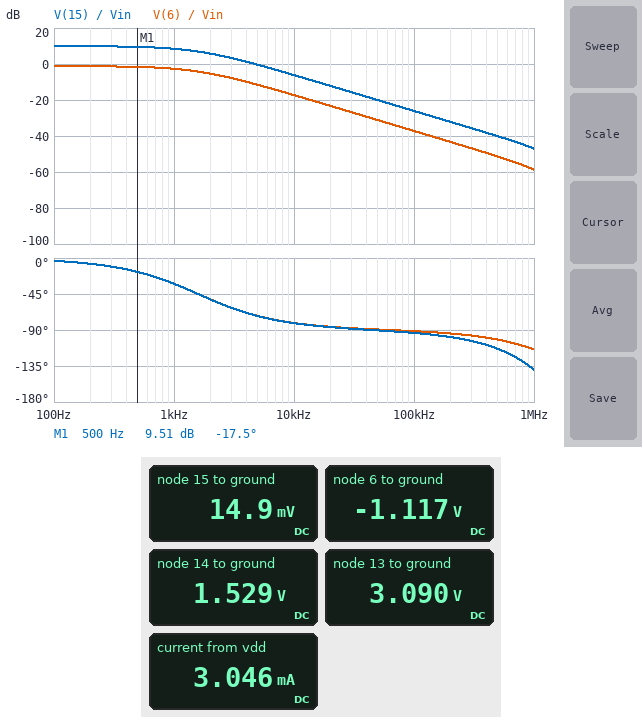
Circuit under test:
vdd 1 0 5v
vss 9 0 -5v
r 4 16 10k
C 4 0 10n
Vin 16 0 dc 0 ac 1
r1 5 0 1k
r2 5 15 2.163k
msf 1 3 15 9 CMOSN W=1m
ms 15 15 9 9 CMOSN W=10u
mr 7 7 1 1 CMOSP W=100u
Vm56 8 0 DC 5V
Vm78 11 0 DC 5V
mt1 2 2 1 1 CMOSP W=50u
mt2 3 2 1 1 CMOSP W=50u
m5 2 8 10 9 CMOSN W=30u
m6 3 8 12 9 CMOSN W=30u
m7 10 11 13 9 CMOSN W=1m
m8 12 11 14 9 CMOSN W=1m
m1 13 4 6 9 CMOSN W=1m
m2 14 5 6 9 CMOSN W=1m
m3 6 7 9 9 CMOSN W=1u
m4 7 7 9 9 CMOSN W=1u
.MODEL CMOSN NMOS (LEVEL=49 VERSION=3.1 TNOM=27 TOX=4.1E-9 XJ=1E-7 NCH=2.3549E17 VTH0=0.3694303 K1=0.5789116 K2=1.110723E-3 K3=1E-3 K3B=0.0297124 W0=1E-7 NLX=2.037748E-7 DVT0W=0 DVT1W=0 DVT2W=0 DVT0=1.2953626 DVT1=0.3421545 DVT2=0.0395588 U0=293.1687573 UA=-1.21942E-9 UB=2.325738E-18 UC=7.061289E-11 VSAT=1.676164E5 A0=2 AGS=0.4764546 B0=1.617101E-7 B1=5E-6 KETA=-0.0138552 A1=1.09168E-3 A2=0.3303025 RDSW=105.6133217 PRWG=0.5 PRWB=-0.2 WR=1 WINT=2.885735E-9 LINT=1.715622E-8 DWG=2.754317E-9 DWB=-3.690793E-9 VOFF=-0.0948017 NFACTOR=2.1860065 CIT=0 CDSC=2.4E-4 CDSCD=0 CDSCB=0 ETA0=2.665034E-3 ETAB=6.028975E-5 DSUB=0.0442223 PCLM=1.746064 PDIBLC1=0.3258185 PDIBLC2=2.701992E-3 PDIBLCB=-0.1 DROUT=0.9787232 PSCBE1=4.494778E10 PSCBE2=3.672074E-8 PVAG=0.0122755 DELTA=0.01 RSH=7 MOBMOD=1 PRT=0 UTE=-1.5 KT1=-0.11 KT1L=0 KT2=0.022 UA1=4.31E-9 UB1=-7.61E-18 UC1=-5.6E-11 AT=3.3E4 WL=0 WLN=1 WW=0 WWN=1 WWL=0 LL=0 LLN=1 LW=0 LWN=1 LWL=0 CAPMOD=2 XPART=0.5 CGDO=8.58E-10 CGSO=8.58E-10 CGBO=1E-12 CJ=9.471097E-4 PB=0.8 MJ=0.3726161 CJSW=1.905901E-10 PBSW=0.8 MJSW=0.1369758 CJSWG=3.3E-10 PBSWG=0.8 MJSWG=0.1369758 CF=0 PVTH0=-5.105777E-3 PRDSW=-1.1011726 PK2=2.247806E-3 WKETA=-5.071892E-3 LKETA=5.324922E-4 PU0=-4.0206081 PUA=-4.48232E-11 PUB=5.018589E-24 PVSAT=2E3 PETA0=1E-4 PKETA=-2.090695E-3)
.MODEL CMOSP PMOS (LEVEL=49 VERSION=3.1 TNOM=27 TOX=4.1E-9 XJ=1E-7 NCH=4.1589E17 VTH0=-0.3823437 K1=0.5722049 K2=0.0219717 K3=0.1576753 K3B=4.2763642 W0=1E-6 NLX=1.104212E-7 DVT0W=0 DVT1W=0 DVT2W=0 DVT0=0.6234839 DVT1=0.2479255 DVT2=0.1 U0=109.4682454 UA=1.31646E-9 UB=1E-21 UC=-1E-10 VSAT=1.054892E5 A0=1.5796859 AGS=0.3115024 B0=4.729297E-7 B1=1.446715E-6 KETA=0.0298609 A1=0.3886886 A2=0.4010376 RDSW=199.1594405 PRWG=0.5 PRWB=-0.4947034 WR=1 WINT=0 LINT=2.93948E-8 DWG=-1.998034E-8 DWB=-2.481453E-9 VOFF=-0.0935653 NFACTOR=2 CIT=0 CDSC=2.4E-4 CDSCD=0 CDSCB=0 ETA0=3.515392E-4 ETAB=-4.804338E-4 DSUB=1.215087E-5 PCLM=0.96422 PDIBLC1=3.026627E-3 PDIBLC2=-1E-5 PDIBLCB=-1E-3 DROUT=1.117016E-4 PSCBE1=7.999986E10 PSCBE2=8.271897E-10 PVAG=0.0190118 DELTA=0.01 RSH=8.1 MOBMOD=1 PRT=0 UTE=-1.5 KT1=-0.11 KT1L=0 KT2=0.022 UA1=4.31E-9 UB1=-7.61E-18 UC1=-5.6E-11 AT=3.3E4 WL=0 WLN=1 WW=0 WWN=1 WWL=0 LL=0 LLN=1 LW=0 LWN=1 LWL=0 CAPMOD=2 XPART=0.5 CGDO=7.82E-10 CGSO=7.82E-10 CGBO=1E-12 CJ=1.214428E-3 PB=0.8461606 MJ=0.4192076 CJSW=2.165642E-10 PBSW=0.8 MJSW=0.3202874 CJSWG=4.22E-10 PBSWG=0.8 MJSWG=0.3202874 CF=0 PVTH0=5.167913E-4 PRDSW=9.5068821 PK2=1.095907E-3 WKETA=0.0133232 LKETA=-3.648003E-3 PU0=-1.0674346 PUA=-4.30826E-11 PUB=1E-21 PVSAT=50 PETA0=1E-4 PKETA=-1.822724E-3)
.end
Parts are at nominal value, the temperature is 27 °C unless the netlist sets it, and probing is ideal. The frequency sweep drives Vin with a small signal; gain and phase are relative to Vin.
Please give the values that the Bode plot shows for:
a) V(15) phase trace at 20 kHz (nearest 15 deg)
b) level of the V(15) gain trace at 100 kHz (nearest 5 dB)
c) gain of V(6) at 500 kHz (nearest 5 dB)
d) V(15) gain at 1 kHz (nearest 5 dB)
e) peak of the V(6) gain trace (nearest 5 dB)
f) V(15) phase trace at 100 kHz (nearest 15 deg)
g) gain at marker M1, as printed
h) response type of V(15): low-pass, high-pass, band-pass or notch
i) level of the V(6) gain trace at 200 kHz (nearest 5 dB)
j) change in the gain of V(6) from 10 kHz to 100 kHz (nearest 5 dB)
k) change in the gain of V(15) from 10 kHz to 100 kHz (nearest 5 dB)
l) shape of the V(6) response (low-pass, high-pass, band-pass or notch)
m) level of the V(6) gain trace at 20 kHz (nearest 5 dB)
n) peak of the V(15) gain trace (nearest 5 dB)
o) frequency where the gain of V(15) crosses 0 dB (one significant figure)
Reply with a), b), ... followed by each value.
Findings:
a) -90 deg
b) -25 dB
c) -50 dB
d) 10 dB
e) 0 dB
f) -90 deg
g) 9.51 dB
h) low-pass
i) -45 dB
j) -20 dB
k) -20 dB
l) low-pass
m) -25 dB
n) 10 dB
o) 5 kHz
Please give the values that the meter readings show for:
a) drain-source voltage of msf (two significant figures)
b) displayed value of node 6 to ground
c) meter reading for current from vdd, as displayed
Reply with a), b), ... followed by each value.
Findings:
a) 5.0 V
b) -1.117 V
c) 3.046 mA
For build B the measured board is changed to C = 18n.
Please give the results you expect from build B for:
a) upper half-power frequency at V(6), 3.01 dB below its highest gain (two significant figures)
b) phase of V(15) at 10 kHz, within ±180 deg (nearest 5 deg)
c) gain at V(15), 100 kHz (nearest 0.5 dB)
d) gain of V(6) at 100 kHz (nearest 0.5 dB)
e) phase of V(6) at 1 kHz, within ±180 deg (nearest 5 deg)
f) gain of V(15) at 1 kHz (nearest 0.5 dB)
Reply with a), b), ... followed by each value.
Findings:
a) 880 Hz
b) -85 deg
c) -31.0 dB
d) -42.5 dB
e) -50 deg
f) 6.5 dB
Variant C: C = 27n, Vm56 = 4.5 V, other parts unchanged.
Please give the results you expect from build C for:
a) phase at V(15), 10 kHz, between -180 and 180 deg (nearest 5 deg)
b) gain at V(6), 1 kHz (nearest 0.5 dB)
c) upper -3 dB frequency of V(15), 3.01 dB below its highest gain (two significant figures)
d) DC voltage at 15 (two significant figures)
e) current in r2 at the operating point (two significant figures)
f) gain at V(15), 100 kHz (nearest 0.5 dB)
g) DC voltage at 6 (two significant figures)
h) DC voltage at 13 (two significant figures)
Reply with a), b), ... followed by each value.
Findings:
a) -85 deg
b) -7.0 dB
c) 590 Hz
d) 12 mV
e) 3.9 µA
f) -34.5 dB
g) -1.1 V
h) 2.6 V
